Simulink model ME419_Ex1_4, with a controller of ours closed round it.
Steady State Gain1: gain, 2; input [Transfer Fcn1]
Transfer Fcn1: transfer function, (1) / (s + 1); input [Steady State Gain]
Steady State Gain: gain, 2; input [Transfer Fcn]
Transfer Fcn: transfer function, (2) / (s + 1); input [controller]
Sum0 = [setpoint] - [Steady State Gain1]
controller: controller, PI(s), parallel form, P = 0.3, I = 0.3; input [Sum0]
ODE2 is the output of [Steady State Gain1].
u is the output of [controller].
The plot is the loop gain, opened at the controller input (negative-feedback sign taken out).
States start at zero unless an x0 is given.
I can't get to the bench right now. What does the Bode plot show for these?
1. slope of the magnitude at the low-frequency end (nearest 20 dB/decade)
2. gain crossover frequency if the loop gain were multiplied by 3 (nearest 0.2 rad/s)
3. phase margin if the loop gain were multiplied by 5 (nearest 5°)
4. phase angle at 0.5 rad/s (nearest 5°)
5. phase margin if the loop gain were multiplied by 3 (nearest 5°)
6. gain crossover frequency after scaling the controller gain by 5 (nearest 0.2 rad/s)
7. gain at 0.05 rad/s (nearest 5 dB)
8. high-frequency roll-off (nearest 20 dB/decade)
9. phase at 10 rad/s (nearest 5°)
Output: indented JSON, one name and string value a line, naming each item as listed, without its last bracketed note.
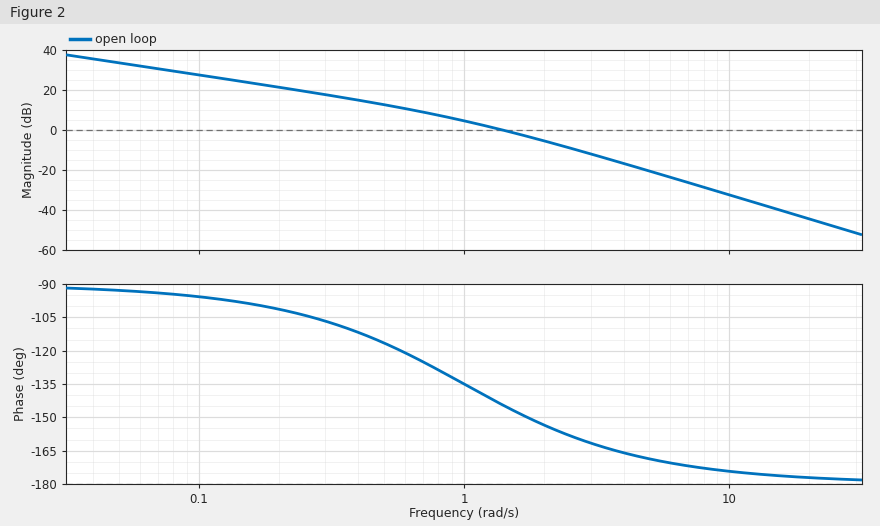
{
  "slope of the magnitude at the low-frequency end": "-20 dB/decade",
  "gain crossover frequency if the loop gain were multiplied by 3": "2.6 rad/s",
  "phase margin if the loop gain were multiplied by 5": "15°",
  "phase angle at 0.5 rad/s": "-115°",
  "phase margin if the loop gain were multiplied by 3": "20°",
  "gain crossover frequency after scaling the controller gain by 5": "3.4 rad/s",
  "gain at 0.05 rad/s": "35 dB",
  "high-frequency roll-off": "-40 dB/decade",
  "phase at 10 rad/s": "-175°"
}
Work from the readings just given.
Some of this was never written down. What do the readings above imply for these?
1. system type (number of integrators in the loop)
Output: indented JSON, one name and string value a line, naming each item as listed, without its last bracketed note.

{
  "system type": "1"
}
